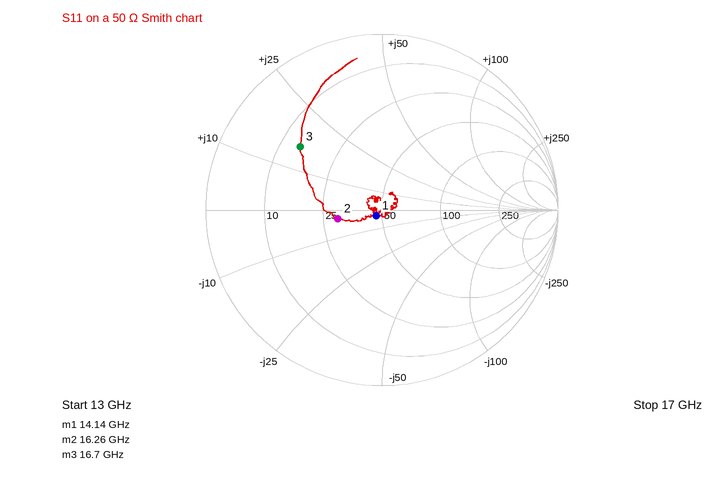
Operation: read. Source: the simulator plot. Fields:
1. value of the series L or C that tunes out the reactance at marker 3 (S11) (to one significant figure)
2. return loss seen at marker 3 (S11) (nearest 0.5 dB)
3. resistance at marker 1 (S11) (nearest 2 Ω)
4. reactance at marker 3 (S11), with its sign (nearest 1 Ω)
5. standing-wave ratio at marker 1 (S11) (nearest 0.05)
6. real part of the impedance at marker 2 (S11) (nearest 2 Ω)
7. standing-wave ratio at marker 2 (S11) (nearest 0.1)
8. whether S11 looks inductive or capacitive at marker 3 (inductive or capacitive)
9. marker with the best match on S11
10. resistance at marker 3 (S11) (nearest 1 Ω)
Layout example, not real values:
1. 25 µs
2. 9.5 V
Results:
1. 600 fF
2. 4.5 dB
3. 46 Ω
4. +16 Ω
5. 1.10
6. 30 Ω
7. 1.7
8. inductive
9. marker 1
10. 14 Ω
